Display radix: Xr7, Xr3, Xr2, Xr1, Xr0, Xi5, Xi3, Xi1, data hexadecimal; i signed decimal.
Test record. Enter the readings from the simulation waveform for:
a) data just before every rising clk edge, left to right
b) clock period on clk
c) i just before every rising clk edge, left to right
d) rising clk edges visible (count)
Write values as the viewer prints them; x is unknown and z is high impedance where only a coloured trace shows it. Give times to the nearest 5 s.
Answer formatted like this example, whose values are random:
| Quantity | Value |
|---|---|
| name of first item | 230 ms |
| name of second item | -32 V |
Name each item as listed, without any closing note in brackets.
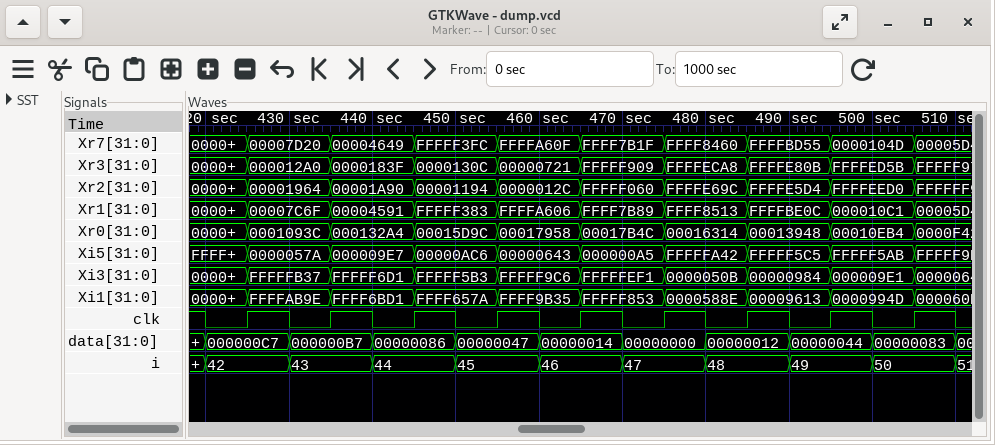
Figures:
| Quantity | Value |
|---|---|
| data just before every rising clk edge, left to right | 000000C7, 000000B7, 00000086, 00000047, 00000014, 00000000, 00000012, 00000044, 00000083 |
| clock period on clk | 10 s |
| i just before every rising clk edge, left to right | 42, 43, 44, 45, 46, 47, 48, 49, 50 |
| rising clk edges visible | 9 |
